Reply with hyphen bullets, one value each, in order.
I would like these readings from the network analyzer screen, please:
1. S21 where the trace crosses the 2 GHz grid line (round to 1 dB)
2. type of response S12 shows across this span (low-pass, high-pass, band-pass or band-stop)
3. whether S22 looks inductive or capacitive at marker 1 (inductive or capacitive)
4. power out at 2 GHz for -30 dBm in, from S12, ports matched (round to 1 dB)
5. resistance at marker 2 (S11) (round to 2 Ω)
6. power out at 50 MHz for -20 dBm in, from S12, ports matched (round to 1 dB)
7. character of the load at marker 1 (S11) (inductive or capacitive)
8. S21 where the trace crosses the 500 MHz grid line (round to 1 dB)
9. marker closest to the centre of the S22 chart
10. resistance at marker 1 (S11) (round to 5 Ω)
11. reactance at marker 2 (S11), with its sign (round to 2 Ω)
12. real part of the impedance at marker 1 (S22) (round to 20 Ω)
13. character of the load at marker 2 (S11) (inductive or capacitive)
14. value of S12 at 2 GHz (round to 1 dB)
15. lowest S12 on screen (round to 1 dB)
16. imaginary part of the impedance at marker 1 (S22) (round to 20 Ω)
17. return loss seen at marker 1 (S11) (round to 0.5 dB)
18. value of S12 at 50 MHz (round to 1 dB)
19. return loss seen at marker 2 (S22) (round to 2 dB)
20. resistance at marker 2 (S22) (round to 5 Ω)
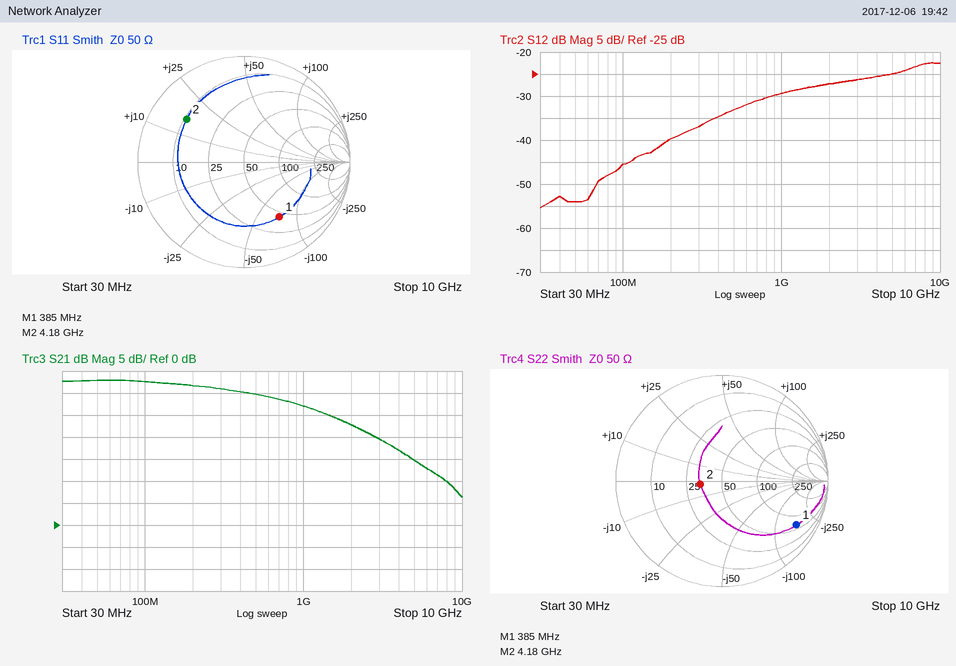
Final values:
- 23 dB
- high-pass
- capacitive
- -57 dBm
- 10 Ω
- -74 dBm
- capacitive
- 30 dB
- marker 2
- 45 Ω
- +16 Ω
- 60 Ω
- inductive
- -27 dB
- -55 dB
- -160 Ω
- 4.0 dB
- -54 dB
- 14 dB
- 35 Ω
